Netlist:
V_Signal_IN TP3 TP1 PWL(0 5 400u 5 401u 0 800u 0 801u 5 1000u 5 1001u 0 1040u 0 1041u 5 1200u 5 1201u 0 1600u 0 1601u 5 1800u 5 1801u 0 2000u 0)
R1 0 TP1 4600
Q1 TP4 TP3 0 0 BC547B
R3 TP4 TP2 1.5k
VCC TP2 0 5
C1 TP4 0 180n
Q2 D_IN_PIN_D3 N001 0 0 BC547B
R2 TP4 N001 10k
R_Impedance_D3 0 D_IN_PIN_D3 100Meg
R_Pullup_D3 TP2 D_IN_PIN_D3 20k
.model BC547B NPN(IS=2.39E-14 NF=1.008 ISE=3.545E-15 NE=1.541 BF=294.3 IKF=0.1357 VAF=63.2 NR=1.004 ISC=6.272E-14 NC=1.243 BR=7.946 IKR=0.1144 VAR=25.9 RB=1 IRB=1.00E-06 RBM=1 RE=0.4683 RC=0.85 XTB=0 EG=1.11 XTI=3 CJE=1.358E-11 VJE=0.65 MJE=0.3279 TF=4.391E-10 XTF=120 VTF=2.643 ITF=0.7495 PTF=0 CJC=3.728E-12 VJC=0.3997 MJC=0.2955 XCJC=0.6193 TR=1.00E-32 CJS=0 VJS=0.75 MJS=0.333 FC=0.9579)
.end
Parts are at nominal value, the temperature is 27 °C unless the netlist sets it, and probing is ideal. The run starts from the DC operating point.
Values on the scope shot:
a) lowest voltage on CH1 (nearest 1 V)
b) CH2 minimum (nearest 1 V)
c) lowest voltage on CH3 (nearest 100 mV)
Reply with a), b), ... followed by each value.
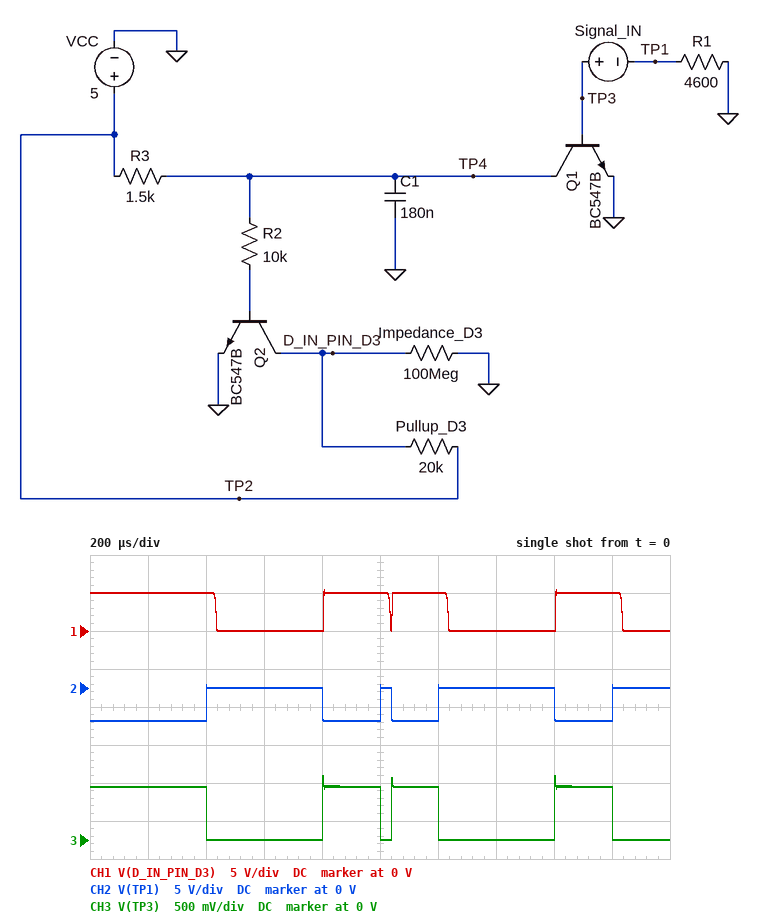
a) 0 V
b) -4 V
c) 0 V
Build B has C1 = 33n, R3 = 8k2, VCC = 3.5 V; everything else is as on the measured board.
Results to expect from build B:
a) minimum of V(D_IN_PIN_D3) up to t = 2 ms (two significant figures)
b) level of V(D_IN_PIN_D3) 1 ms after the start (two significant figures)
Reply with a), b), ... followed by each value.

a) 11 mV
b) 3.5 V
